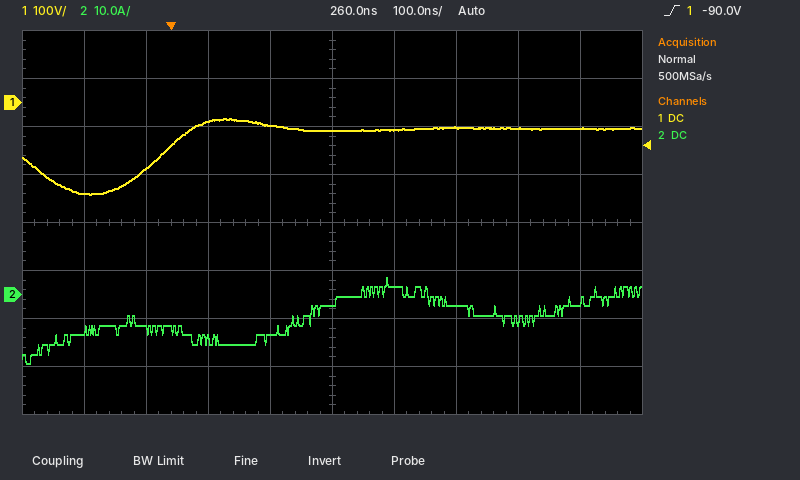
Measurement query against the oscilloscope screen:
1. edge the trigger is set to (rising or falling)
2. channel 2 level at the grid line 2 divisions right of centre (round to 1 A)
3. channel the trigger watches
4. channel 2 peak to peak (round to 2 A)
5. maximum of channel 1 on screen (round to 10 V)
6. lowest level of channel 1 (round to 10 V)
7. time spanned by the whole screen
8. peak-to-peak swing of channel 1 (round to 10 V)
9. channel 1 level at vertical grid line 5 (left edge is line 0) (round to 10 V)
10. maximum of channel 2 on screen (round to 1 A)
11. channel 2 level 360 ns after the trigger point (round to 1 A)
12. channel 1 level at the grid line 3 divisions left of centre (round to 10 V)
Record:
rising
-2 A
channel 1
18 A
-30 V
-190 V
1 µs
160 V
-60 V
4 A
2 A
-140 V
